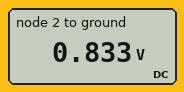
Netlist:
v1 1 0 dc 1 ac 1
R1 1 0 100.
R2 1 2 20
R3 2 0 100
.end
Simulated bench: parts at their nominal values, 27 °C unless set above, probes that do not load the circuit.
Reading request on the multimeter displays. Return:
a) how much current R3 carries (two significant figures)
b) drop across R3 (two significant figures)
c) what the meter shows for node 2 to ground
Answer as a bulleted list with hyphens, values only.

- 8.3 mA
- 830 mV
- 0.833 V
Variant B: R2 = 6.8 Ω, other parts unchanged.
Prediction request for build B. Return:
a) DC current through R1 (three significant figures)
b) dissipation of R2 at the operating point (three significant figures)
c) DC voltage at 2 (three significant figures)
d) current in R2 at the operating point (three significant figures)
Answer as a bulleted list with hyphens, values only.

- 10.0 mA
- 596 µW
- 936 mV
- 9.36 mA
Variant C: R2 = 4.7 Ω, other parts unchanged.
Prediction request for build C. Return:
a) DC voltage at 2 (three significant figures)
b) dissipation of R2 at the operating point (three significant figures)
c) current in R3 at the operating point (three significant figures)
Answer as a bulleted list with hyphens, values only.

- 955 mV
- 429 µW
- 9.55 mA
